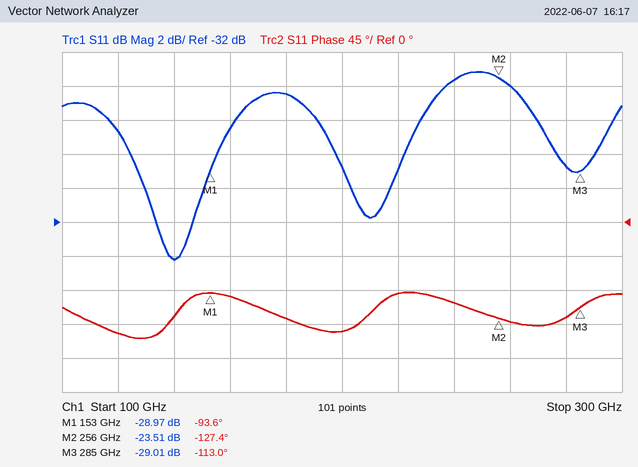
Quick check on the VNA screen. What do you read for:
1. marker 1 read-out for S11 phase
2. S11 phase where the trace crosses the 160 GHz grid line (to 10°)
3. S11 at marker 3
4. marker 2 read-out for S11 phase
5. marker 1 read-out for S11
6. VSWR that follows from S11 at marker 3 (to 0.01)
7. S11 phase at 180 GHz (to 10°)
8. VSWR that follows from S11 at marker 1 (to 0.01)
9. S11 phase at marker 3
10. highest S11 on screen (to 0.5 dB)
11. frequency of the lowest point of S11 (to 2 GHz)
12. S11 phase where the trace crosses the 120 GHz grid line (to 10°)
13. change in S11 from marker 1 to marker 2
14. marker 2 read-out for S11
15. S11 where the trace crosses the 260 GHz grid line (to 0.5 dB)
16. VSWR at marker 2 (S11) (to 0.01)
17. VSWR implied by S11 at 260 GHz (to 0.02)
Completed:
-93.6°
-100°
-29.01 dB
-127.4°
-28.97 dB
1.07
-130°
1.07
-113.0°
-23.0 dB
140 GHz
-150°
5.46 dB
-23.51 dB
-24.0 dB
1.14
1.14
